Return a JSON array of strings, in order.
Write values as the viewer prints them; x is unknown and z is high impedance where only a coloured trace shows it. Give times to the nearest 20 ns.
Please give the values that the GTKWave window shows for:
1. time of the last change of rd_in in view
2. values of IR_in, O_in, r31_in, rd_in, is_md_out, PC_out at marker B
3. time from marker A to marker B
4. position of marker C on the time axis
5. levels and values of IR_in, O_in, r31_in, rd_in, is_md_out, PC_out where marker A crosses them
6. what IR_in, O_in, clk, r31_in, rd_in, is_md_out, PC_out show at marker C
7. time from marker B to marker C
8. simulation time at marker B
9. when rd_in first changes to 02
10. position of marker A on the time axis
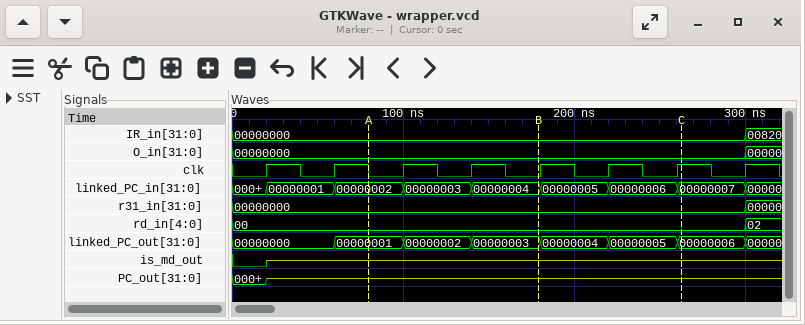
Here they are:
["300 ns", "IR_in=00000000, O_in=00000000, r31_in=00000000, rd_in=00, is_md_out=z, PC_out=z", "100 ns", "260 ns", "IR_in=00000000, O_in=00000000, r31_in=00000000, rd_in=00, is_md_out=z, PC_out=z", "IR_in=00000000, O_in=00000000, clk=1, r31_in=00000000, rd_in=00, is_md_out=z, PC_out=z", "80 ns", "180 ns", "300 ns", "80 ns"]
